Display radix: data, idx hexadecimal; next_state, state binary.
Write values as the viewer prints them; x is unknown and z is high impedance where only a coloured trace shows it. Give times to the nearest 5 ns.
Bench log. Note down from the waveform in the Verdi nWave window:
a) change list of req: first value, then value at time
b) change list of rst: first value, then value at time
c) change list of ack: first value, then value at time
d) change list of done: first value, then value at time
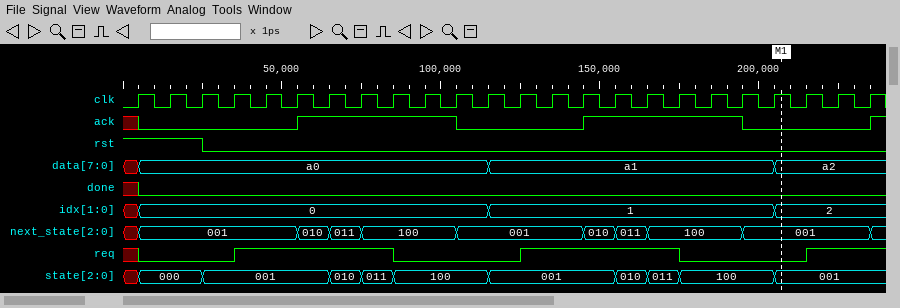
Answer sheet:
x, 0 at 5 ns, 1 at 35 ns, 0 at 85 ns, 1 at 125 ns, 0 at 175 ns, 1 at 215 ns
1, 0 at 25 ns
x, 0 at 5 ns, 1 at 55 ns, 0 at 105 ns, 1 at 145 ns, 0 at 195 ns, 1 at 235 ns
x, 0 at 5 ns
